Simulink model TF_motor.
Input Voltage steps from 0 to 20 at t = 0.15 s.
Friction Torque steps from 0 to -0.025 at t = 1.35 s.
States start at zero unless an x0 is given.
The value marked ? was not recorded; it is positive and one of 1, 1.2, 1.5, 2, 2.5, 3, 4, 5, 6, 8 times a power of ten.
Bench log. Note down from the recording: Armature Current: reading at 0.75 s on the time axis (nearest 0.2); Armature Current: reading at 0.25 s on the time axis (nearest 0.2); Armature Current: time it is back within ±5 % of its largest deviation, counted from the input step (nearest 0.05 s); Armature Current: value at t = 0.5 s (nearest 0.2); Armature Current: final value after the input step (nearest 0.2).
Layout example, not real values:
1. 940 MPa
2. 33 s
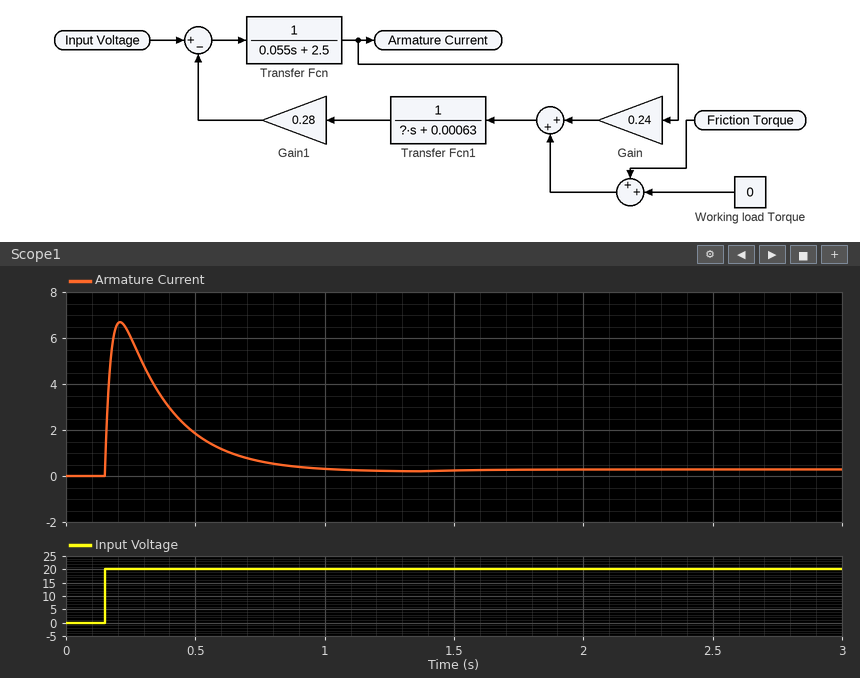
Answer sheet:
1. 0.6
2. 6.0
3. 0.65 s
4. 1.8
5. 0.2
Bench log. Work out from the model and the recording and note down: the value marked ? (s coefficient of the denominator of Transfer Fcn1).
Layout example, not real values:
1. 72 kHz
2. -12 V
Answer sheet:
1. 0.006
